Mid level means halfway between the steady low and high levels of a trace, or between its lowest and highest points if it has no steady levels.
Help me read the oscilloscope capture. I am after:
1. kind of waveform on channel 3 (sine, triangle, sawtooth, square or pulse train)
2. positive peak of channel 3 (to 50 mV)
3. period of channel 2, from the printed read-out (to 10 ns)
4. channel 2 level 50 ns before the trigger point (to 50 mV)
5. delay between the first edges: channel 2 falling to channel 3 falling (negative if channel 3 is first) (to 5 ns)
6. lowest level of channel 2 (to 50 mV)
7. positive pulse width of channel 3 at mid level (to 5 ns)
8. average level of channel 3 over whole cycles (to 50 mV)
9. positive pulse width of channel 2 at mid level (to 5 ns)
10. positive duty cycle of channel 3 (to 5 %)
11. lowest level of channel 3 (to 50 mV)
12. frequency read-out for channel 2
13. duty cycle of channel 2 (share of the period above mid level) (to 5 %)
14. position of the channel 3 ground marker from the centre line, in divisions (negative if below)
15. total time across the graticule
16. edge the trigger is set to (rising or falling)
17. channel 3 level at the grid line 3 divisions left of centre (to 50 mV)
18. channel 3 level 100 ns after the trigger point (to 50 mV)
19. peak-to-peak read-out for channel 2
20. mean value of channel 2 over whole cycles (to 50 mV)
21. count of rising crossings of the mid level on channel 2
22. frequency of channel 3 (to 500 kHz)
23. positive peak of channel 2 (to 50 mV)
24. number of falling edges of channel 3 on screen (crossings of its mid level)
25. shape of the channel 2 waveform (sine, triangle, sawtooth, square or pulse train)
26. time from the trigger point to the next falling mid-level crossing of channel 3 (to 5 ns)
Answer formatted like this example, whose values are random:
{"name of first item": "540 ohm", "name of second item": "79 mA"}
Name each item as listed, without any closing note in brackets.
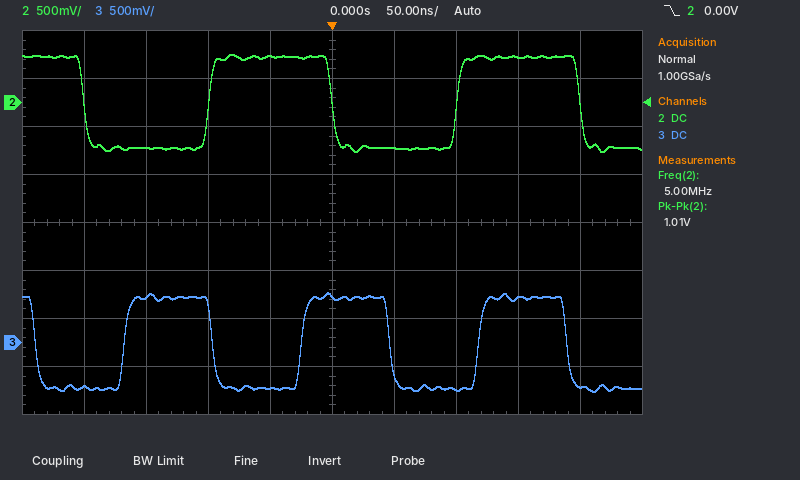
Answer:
{"kind of waveform on channel 3": "square", "positive peak of channel 3": "500 mV", "period of channel 2, from the printed read-out": "200 ns", "channel 2 level 50 ns before the trigger point": "500 mV", "delay between the first edges: channel 2 falling to channel 3 falling (negative if channel 3 is first)": "-40 ns", "lowest level of channel 2": "-500 mV", "positive pulse width of channel 3 at mid level": "70 ns", "average level of channel 3 over whole cycles": "0 mV", "positive pulse width of channel 2 at mid level": "100 ns", "positive duty cycle of channel 3": "50 %", "lowest level of channel 3": "-500 mV", "frequency read-out for channel 2": "5.00 MHz", "duty cycle of channel 2 (share of the period above mid level)": "50 %", "position of the channel 3 ground marker from the centre line, in divisions": "-2.5 div", "total time across the graticule": "500 ns", "edge the trigger is set to": "falling", "channel 3 level at the grid line 3 divisions left of centre": "500 mV", "channel 3 level 100 ns after the trigger point": "-500 mV", "peak-to-peak read-out for channel 2": "1.01 V", "mean value of channel 2 over whole cycles": "0 mV", "count of rising crossings of the mid level on channel 2": "2", "frequency of channel 3": "7.0 MHz", "positive peak of channel 2": "500 mV", "number of falling edges of channel 3 on screen": "4", "shape of the channel 2 waveform": "square", "time from the trigger point to the next falling mid-level crossing of channel 3": "45 ns"}
